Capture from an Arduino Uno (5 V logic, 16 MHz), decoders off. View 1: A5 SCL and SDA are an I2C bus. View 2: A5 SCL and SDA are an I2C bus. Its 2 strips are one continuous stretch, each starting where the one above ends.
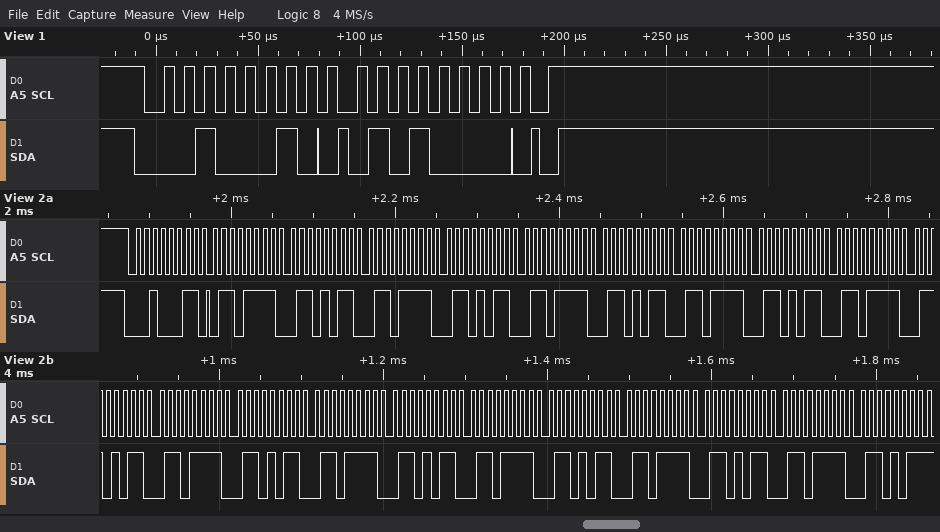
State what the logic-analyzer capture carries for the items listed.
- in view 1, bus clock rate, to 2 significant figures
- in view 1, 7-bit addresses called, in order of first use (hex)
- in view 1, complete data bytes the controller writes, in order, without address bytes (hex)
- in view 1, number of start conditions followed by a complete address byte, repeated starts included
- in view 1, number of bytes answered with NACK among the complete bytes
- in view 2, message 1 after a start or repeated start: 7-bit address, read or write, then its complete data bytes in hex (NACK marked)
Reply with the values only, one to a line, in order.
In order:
100 kHz
0x11
50
1
0
0x11 read: 6F 6B 6F 6B 6F 6B 6F 6B 6F 6B 6F 6B 6F 6B 6F 6B 6F 6B 6F 6B NACK
